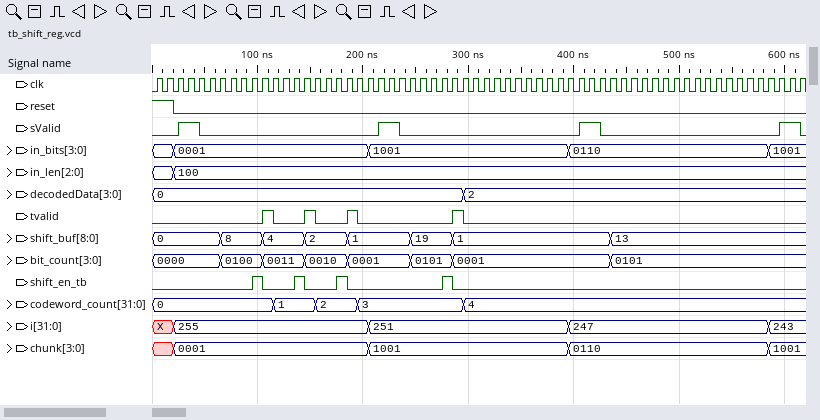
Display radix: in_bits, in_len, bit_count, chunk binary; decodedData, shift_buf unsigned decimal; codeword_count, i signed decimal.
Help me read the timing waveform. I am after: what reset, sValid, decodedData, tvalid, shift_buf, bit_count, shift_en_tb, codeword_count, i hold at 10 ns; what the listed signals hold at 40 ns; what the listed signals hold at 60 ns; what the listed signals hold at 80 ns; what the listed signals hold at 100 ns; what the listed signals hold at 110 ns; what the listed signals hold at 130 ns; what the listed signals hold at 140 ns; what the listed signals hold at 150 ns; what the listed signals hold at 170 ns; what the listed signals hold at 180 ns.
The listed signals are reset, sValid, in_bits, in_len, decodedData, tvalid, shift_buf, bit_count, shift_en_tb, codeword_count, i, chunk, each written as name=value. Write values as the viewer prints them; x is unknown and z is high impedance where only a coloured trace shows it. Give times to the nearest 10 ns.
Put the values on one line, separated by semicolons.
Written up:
reset=1, sValid=0, decodedData=0, tvalid=0, shift_buf=0, bit_count=0000, shift_en_tb=0, codeword_count=0, i=X; reset=0, sValid=1, in_bits=0001, in_len=100, decodedData=0, tvalid=0, shift_buf=0, bit_count=0000, shift_en_tb=0, codeword_count=0, i=255, chunk=0001; reset=0, sValid=0, in_bits=0001, in_len=100, decodedData=0, tvalid=0, shift_buf=0, bit_count=0000, shift_en_tb=0, codeword_count=0, i=255, chunk=0001; reset=0, sValid=0, in_bits=0001, in_len=100, decodedData=0, tvalid=0, shift_buf=8, bit_count=0100, shift_en_tb=0, codeword_count=0, i=255, chunk=0001; reset=0, sValid=0, in_bits=0001, in_len=100, decodedData=0, tvalid=0, shift_buf=8, bit_count=0100, shift_en_tb=1, codeword_count=0, i=255, chunk=0001; reset=0, sValid=0, in_bits=0001, in_len=100, decodedData=0, tvalid=1, shift_buf=4, bit_count=0011, shift_en_tb=0, codeword_count=0, i=255, chunk=0001; reset=0, sValid=0, in_bits=0001, in_len=100, decodedData=0, tvalid=0, shift_buf=4, bit_count=0011, shift_en_tb=0, codeword_count=1, i=255, chunk=0001; reset=0, sValid=0, in_bits=0001, in_len=100, decodedData=0, tvalid=0, shift_buf=4, bit_count=0011, shift_en_tb=1, codeword_count=1, i=255, chunk=0001; reset=0, sValid=0, in_bits=0001, in_len=100, decodedData=0, tvalid=1, shift_buf=2, bit_count=0010, shift_en_tb=0, codeword_count=1, i=255, chunk=0001; reset=0, sValid=0, in_bits=0001, in_len=100, decodedData=0, tvalid=0, shift_buf=2, bit_count=0010, shift_en_tb=0, codeword_count=2, i=255, chunk=0001; reset=0, sValid=0, in_bits=0001, in_len=100, decodedData=0, tvalid=0, shift_buf=2, bit_count=0010, shift_en_tb=1, codeword_count=2, i=255, chunk=0001
